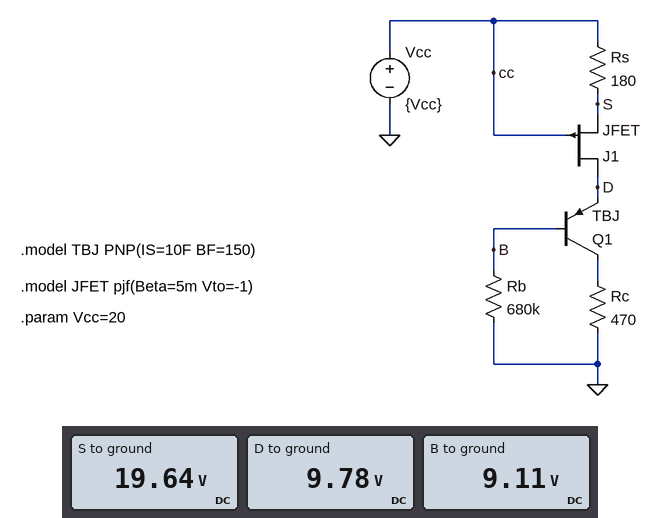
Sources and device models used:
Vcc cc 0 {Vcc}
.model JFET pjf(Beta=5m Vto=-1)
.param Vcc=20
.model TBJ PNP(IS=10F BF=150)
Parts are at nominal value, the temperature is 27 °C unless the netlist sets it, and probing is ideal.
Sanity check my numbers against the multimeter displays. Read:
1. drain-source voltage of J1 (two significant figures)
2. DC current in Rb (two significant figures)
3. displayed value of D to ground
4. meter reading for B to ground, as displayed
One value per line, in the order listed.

-9.9 V
13 µA
9.78 V
9.11 V
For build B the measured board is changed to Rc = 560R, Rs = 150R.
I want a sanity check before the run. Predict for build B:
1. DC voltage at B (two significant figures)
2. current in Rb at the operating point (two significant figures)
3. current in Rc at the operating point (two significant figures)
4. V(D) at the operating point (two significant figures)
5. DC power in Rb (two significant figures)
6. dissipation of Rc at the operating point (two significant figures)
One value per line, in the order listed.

10 V
15 µA
2.2 mA
11 V
150 µW
2.7 mW
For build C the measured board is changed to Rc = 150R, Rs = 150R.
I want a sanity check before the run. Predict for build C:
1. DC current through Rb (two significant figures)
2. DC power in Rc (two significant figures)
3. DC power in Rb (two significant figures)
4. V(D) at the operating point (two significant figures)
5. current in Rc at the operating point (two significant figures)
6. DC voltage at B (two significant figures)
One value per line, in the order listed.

15 µA
730 µW
150 µW
11 V
2.2 mA
10 V
